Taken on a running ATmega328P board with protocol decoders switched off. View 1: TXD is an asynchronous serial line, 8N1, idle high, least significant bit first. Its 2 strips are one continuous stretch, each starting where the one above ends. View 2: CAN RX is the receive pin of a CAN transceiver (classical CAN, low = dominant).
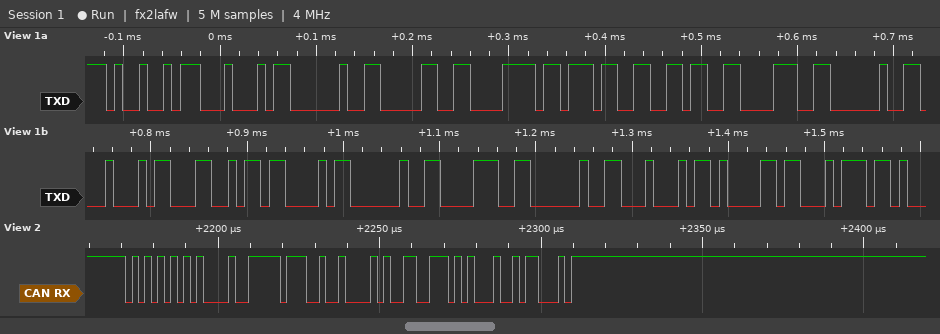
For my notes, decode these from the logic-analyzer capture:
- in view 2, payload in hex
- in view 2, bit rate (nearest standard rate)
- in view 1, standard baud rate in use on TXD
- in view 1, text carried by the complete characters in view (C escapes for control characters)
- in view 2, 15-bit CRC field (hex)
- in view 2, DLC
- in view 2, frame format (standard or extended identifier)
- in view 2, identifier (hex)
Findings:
FF 24 29 9D
500 kbit/s
115200 baud
"ID 0x768 DLC 8 Dat"
0x2258
4
standard
0x555
